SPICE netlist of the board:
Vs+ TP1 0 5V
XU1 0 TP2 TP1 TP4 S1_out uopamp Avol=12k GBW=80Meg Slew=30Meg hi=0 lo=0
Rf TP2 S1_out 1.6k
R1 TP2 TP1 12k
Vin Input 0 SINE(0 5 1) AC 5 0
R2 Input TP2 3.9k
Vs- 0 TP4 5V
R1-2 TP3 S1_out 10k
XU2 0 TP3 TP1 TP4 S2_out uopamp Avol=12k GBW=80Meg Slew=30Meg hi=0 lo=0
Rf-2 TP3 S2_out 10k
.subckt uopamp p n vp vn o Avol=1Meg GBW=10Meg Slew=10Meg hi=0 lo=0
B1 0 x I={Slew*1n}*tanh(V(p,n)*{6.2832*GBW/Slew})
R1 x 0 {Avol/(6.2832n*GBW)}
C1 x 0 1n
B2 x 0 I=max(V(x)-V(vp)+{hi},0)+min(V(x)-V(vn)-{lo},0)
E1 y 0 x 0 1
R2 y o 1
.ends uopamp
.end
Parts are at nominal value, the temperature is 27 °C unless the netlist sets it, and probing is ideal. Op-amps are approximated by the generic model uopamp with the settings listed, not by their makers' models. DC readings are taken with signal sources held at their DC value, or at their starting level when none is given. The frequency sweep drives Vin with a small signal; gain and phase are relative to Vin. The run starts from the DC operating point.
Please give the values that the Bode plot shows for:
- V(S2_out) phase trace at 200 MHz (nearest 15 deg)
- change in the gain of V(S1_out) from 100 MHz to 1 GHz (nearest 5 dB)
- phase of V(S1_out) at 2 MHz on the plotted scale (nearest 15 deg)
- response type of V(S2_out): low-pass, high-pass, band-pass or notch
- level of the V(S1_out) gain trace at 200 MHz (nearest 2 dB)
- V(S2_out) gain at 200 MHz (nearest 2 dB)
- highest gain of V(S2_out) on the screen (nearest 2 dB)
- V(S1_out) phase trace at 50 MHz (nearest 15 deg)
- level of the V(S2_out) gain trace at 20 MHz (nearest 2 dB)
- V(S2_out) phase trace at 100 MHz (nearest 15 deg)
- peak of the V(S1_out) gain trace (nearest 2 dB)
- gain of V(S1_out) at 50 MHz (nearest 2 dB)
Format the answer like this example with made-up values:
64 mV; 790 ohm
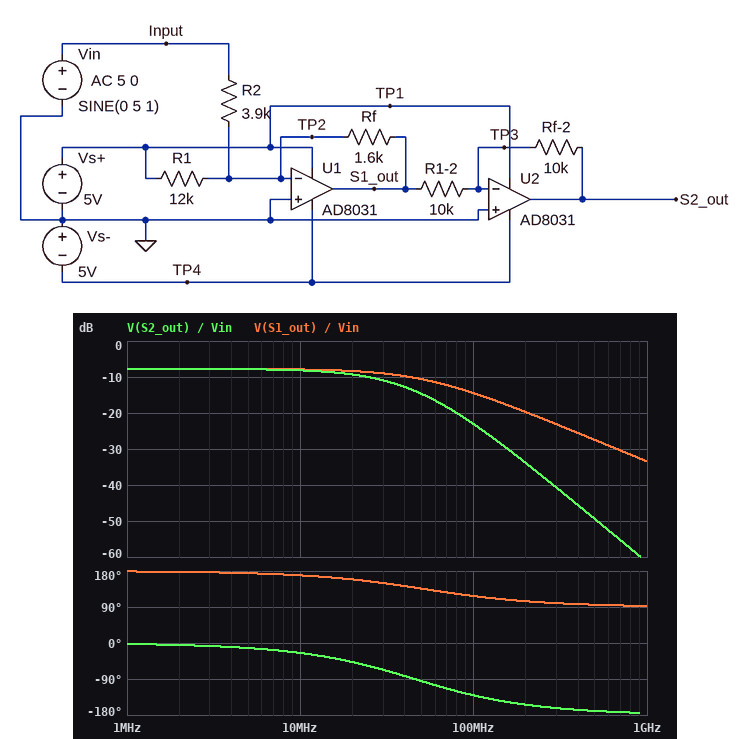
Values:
-150 deg; -20 dB; 180 deg; low-pass; -20 dB; -34 dB; -8 dB; 135 deg; -10 dB; -135 deg; -8 dB; -10 dB
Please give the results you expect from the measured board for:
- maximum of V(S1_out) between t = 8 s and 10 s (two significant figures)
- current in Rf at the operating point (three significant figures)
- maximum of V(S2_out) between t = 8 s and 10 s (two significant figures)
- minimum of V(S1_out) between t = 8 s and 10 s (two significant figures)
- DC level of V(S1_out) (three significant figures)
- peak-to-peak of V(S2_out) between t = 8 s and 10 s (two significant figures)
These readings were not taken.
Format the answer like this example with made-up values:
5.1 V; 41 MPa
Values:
1.4 V; 417 µA; 2.7 V; -2.7 V; -667 mV; 4.1 V
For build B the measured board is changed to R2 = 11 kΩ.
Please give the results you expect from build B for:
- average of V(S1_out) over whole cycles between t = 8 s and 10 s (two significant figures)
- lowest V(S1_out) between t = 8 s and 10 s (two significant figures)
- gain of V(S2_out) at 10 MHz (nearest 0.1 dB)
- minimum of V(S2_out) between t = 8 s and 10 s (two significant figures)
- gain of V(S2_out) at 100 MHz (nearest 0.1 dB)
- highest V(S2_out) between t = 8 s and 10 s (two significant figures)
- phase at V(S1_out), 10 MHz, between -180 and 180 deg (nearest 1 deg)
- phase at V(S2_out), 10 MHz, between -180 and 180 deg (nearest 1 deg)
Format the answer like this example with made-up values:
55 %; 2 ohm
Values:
-670 mV; -1.4 V; -17.1 dB; -61 mV; -30.9 dB; 1.4 V; 171 deg; -23 deg
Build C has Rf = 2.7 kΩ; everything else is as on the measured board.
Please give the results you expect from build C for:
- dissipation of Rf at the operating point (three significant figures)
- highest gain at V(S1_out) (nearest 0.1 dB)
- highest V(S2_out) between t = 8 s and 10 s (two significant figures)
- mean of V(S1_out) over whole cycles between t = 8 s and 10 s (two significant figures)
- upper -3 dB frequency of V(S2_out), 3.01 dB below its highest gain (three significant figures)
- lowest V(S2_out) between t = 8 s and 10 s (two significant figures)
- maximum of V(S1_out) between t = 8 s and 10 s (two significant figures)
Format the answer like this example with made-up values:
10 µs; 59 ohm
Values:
469 µW; -3.2 dB; 4.6 V; -1.1 V; 26.3 MHz; -2.3 V; 2.3 V
